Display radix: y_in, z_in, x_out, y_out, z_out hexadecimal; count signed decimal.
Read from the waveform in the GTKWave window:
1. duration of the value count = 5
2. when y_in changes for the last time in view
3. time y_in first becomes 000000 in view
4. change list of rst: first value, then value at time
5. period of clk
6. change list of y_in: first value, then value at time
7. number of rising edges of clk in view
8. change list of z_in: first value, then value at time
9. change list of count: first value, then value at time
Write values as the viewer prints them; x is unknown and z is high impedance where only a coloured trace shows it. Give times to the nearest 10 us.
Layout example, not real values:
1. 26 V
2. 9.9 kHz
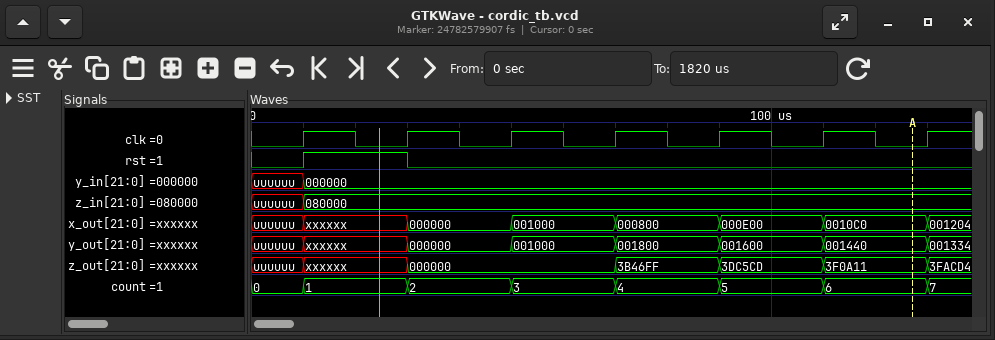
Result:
1. 20 us
2. 10 us
3. 10 us
4. 0, 1 at 10 us, 0 at 30 us
5. 20 us
6. uuuuuu, 000000 at 10 us
7. 7
8. uuuuuu, 080000 at 10 us
9. 0, 1 at 10 us, 2 at 30 us, 3 at 50 us, 4 at 70 us, 5 at 90 us, 6 at 110 us, 7 at 130 us
